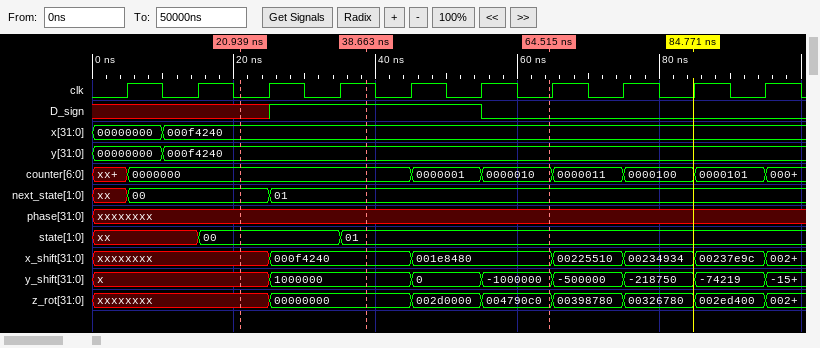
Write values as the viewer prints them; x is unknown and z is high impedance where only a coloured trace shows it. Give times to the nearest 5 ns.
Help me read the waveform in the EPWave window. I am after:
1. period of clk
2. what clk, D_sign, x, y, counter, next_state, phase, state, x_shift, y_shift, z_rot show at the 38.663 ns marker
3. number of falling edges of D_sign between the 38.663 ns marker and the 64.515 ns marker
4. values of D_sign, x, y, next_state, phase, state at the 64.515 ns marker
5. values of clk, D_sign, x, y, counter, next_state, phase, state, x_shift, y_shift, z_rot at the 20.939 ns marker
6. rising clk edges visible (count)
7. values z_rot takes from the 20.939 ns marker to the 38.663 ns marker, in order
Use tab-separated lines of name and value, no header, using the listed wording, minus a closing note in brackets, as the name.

period of clk	10 ns
what clk, D_sign, x, y, counter, next_state, phase, state, x_shift, y_shift, z_rot show at the 38.663 ns marker	clk=1, D_sign=1, x=000f4240, y=000f4240, counter=0000000, next_state=01, phase=xxxxxxxx, state=01, x_shift=000f4240, y_shift=1000000, z_rot=00000000
number of falling edges of D_sign between the 38.663 ns marker and the 64.515 ns marker	1
values of D_sign, x, y, next_state, phase, state at the 64.515 ns marker	D_sign=0, x=000f4240, y=000f4240, next_state=01, phase=xxxxxxxx, state=01
values of clk, D_sign, x, y, counter, next_state, phase, state, x_shift, y_shift, z_rot at the 20.939 ns marker	clk=0, D_sign=x, x=000f4240, y=000f4240, counter=0000000, next_state=00, phase=xxxxxxxx, state=00, x_shift=xxxxxxxx, y_shift=x, z_rot=xxxxxxxx
rising clk edges visible	10
values z_rot takes from the 20.939 ns marker to the 38.663 ns marker, in order	xxxxxxxx, 00000000
